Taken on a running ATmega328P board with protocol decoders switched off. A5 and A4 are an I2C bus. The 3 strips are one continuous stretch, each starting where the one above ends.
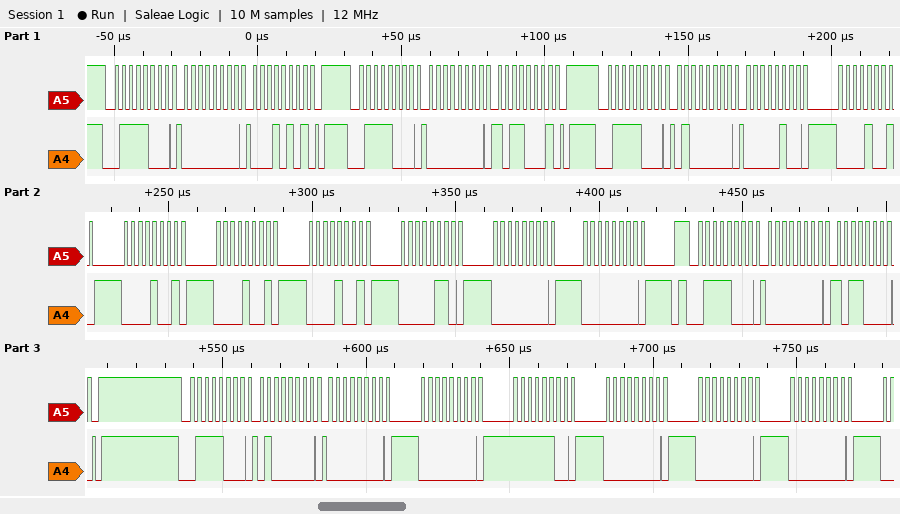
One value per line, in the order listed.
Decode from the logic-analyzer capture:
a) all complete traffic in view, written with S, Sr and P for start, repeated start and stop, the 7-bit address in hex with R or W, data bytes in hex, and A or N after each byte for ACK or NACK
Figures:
S 3CW A 00 A 15 A P S 3CW A 00 A B1 A P S 3CW A 40 A 04 A 09 A 09 A 09 A 09 A 06 A 00 A 00 A P S 3CW A 00 A B0 A P S 3CW A 40 A 00 A 00 A FC A 00 A 00 A 00 A
